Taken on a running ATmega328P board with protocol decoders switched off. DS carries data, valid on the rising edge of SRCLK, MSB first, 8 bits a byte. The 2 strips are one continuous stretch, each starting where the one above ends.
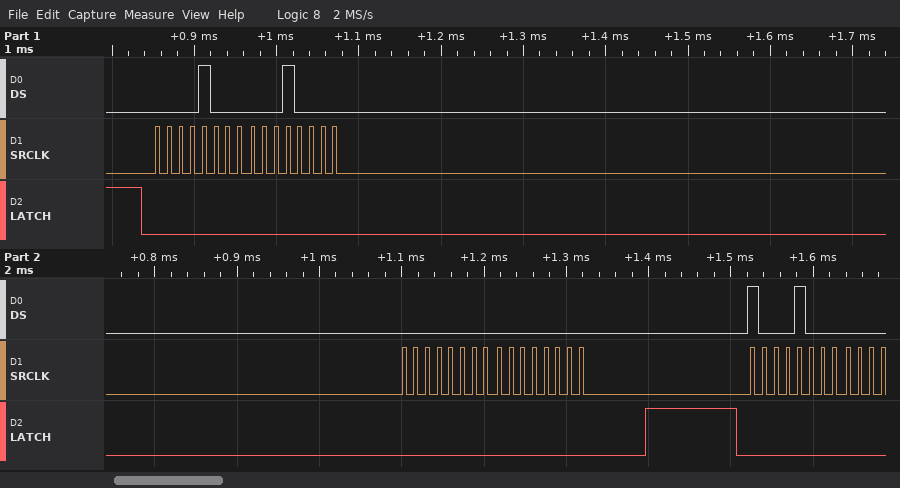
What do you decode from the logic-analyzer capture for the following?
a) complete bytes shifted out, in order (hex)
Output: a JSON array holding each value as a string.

["0x08 0x10 0x00 0x00 0x88"]
